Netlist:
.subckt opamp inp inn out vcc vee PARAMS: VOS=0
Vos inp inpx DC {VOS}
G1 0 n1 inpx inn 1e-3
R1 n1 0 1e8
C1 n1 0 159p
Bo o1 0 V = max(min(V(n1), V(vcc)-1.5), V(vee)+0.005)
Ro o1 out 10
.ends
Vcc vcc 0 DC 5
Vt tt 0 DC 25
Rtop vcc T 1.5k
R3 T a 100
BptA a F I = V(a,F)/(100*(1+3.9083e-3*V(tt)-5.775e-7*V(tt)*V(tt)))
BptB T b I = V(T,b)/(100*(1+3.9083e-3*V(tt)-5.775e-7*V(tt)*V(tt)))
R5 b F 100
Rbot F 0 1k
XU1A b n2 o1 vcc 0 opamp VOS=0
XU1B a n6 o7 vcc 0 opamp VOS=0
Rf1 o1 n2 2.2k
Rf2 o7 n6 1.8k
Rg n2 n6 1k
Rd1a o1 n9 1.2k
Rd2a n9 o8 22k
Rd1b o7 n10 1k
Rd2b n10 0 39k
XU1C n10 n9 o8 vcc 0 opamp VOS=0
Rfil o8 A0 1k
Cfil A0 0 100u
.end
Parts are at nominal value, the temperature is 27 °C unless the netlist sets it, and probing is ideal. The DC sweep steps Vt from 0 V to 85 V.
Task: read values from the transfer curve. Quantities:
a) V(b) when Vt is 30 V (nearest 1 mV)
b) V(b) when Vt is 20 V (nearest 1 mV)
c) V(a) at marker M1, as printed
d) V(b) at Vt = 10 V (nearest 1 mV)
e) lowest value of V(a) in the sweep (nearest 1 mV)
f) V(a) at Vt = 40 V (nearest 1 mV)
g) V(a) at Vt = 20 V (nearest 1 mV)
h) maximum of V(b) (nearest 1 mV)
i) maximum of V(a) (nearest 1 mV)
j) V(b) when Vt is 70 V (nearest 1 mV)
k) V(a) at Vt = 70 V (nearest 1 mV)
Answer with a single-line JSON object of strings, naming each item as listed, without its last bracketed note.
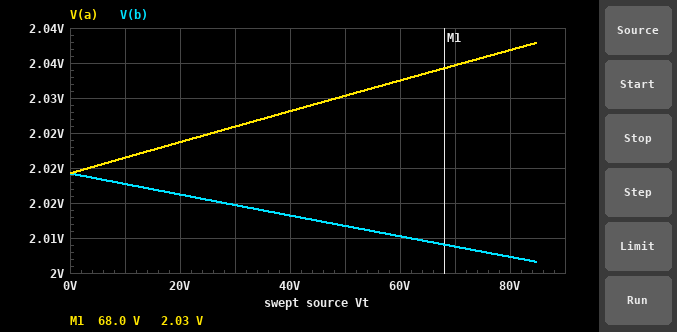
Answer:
{"V(b) when Vt is 30 V": "2.015 V", "V(b) when Vt is 20 V": "2.016 V", "V(a) at marker M1, as printed": "2.03 V", "V(b) at Vt = 10 V": "2.018 V", "lowest value of V(a) in the sweep": "2.019 V", "V(a) at Vt = 40 V": "2.028 V", "V(a) at Vt = 20 V": "2.024 V", "maximum of V(b)": "2.019 V", "maximum of V(a)": "2.038 V", "V(b) when Vt is 70 V": "2.009 V", "V(a) at Vt = 70 V": "2.035 V"}
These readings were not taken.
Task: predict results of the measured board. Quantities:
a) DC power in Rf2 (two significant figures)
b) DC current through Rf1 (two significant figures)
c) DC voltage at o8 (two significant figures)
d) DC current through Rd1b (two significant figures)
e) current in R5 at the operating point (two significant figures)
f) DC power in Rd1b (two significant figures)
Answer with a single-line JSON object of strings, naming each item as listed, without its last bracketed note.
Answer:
{"DC power in Rf2": "160 nW", "DC current through Rf1": "9.3 µA", "DC voltage at o8": "1.9 V", "DC current through Rd1b": "51 µA", "current in R5 at the operating point": "960 µA", "DC power in Rd1b": "2.6 µW"}
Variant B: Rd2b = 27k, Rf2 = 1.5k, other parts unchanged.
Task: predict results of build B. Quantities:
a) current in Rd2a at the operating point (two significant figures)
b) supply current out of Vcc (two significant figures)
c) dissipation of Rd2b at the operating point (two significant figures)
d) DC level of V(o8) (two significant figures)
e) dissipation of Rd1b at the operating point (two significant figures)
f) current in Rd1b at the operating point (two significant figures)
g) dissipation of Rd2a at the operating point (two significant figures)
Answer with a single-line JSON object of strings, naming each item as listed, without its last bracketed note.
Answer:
{"current in Rd2a at the operating point": "24 µA", "supply current out of Vcc": "1.9 mA", "dissipation of Rd2b at the operating point": "140 µW", "DC level of V(o8)": "1.4 V", "dissipation of Rd1b at the operating point": "5.3 µW", "current in Rd1b at the operating point": "73 µA", "dissipation of Rd2a at the operating point": "13 µW"}
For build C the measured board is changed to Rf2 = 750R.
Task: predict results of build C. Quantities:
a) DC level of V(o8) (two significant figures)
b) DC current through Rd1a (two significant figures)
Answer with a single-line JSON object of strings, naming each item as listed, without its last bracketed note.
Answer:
{"DC level of V(o8)": "1.7 V", "DC current through Rd1a": "12 µA"}
